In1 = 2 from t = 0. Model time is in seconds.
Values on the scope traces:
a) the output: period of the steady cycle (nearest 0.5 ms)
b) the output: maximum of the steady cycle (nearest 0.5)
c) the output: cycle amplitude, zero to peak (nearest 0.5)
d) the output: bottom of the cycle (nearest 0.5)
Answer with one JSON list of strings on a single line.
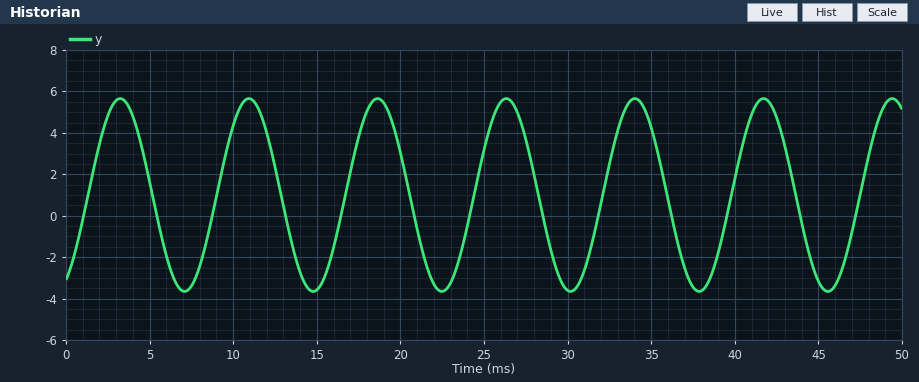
["7.5 ms", "5.5", "4.5", "-3.5"]
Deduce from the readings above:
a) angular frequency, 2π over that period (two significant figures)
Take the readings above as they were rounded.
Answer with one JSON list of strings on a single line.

["0.84 rad/ms"]
